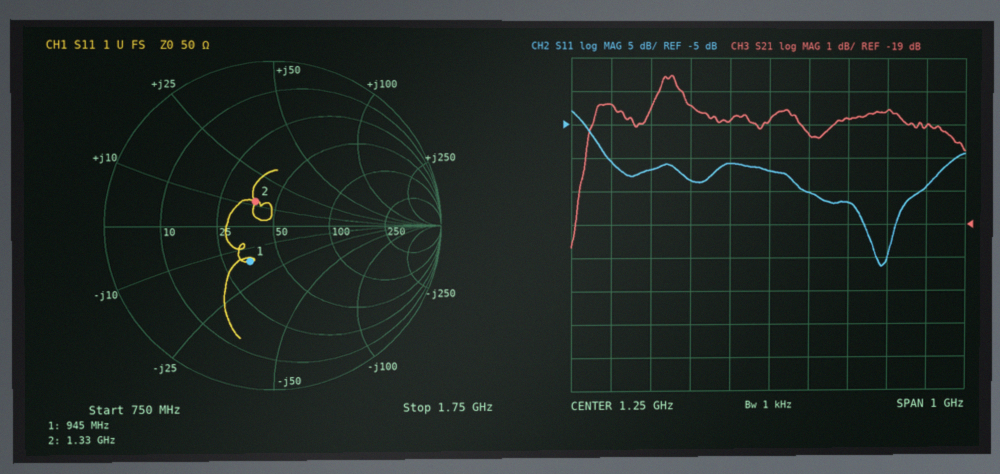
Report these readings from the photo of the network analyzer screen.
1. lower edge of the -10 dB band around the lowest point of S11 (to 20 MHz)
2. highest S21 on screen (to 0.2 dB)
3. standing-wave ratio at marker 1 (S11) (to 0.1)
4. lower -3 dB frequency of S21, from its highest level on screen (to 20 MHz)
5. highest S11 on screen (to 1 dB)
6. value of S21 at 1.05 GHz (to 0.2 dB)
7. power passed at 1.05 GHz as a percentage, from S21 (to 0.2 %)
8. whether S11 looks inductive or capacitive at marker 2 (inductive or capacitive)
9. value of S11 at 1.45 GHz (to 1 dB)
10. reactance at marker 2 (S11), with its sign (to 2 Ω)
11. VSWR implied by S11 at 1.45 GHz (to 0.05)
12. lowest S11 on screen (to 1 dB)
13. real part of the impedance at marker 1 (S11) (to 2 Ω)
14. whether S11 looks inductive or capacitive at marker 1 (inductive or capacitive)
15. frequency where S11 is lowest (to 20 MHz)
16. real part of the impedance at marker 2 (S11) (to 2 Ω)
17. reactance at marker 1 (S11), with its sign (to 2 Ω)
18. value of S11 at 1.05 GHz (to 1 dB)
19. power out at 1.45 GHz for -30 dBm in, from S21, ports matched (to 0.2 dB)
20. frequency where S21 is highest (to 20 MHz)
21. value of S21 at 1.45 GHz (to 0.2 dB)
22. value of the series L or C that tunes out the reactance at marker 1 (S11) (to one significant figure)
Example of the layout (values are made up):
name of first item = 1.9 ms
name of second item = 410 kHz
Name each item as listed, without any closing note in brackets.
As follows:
lower edge of the -10 dB band around the lowest point of S11 = 840 MHz
highest S21 on screen = -14.6 dB
standing-wave ratio at marker 1 (S11) = 1.7
lower -3 dB frequency of S21, from its highest level on screen = 780 MHz
highest S11 on screen = -3 dB
value of S21 at 1.05 GHz = -15.4 dB
power passed at 1.05 GHz as a percentage, from S21 = 2.8 %
whether S11 looks inductive or capacitive at marker 2 = inductive
value of S11 at 1.45 GHz = -17 dB
reactance at marker 2 (S11), with its sign = +12 Ω
VSWR implied by S11 at 1.45 GHz = 1.35
lowest S11 on screen = -26 dB
real part of the impedance at marker 1 (S11) = 34 Ω
whether S11 looks inductive or capacitive at marker 1 = capacitive
frequency where S11 is lowest = 1.54 GHz
real part of the impedance at marker 2 (S11) = 38 Ω
reactance at marker 1 (S11), with its sign = -16 Ω
value of S11 at 1.05 GHz = -13 dB
power out at 1.45 GHz for -30 dBm in, from S21, ports matched = -45.8 dBm
frequency where S21 is highest = 1.00 GHz
value of S21 at 1.45 GHz = -15.8 dB
value of the series L or C that tunes out the reactance at marker 1 (S11) = 3 nH
